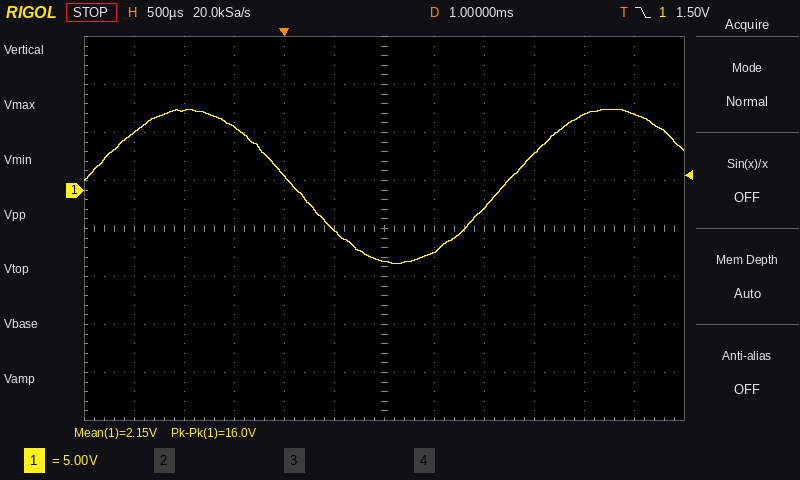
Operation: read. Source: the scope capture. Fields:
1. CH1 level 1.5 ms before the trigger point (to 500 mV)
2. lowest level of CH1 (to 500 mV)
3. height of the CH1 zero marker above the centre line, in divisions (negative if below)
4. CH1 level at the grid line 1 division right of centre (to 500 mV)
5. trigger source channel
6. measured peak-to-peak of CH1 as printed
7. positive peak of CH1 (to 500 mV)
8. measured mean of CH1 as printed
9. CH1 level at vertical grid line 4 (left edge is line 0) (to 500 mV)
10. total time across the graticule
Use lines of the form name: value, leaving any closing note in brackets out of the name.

CH1 level 1.5 ms before the trigger point: 6.0 V
lowest level of CH1: -7.5 V
height of the CH1 zero marker above the centre line, in divisions: +0.8 div
CH1 level at the grid line 1 division right of centre: -6.5 V
trigger source channel: CH1
measured peak-to-peak of CH1 as printed: 16.0 V
positive peak of CH1: 8.5 V
measured mean of CH1 as printed: 2.15 V
CH1 level at vertical grid line 4 (left edge is line 0): 1.5 V
total time across the graticule: 6 ms
